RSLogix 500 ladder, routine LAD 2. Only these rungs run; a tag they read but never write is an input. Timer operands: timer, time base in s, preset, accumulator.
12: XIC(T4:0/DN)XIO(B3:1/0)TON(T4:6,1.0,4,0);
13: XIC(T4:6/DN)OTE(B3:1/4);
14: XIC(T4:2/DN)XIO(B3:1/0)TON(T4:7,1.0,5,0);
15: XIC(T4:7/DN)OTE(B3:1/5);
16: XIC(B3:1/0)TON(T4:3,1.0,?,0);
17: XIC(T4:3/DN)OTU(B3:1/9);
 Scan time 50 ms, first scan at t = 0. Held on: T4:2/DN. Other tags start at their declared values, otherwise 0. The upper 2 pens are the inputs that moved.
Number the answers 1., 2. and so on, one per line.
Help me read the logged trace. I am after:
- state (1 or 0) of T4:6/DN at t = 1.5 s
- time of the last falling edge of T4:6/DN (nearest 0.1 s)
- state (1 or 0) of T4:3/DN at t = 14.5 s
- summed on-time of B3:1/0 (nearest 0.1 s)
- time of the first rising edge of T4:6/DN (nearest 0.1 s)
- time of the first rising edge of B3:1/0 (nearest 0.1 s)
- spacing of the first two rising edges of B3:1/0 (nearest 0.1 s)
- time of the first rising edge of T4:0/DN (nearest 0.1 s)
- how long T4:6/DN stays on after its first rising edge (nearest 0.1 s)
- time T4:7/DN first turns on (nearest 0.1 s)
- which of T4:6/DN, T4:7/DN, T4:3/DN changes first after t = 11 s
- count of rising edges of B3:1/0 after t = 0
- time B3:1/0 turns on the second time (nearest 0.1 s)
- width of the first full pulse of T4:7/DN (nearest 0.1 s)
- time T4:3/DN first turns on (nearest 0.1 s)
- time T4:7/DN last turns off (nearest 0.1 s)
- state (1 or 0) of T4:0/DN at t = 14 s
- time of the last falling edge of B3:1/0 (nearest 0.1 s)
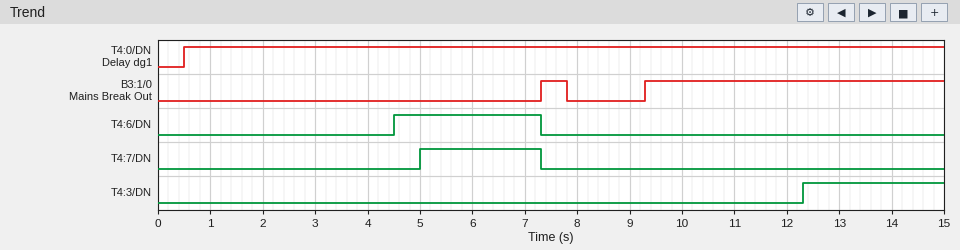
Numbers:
1. 0
2. 7.3 s
3. 1
4. 6.2 s
5. 4.5 s
6. 7.3 s
7. 2.0 s
8. 0.5 s
9. 2.8 s
10. 5.0 s
11. T4:3/DN
12. 2
13. 9.3 s
14. 2.3 s
15. 12.3 s
16. 7.3 s
17. 1
18. 7.8 s
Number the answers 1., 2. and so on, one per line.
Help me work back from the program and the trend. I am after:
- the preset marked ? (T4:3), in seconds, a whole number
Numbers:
1. 3 s
